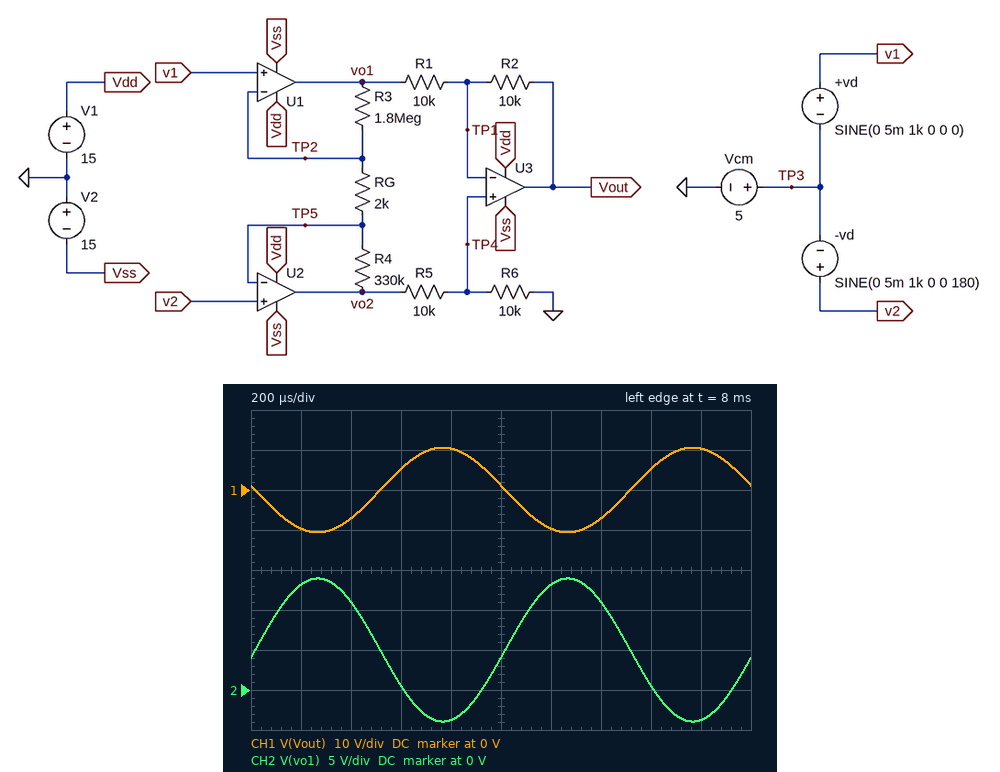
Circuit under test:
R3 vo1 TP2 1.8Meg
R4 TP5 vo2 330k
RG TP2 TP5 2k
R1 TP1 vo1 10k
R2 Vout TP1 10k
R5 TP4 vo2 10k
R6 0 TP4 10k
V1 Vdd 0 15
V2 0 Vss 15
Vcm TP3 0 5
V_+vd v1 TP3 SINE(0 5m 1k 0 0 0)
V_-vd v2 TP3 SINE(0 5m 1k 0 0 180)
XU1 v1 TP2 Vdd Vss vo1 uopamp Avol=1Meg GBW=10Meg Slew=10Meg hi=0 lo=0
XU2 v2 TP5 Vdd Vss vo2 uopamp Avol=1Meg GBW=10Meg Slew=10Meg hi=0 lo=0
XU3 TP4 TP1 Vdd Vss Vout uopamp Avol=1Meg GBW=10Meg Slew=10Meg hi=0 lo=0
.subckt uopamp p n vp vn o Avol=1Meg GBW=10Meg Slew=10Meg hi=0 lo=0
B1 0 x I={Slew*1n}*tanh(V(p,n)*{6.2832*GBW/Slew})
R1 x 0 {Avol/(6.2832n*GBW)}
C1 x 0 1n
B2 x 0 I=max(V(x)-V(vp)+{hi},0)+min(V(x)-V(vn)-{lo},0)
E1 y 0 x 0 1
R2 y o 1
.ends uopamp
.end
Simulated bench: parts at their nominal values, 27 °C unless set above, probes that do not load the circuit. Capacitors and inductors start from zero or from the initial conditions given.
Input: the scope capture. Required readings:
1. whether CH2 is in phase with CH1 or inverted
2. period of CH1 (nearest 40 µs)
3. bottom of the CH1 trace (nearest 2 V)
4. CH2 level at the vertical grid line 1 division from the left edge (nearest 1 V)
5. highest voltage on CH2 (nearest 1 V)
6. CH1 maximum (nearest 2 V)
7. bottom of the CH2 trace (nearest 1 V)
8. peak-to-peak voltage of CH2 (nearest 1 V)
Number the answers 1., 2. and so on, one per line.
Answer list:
1. inverted
2. 1.00 ms
3. -10 V
4. 13 V
5. 14 V
6. 10 V
7. -4 V
8. 18 V
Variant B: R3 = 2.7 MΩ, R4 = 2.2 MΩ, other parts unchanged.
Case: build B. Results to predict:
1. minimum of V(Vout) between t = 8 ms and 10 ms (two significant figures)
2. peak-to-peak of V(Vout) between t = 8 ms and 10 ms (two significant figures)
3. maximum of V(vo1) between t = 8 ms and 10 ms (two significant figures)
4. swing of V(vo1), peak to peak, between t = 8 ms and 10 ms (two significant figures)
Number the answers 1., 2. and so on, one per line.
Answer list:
1. -15 V
2. 30 V
3. 15 V
4. 22 V
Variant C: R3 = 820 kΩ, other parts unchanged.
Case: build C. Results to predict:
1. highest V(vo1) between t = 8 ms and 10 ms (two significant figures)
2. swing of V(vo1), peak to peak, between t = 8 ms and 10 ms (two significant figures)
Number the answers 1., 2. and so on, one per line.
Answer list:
1. 9.1 V
2. 8.2 V
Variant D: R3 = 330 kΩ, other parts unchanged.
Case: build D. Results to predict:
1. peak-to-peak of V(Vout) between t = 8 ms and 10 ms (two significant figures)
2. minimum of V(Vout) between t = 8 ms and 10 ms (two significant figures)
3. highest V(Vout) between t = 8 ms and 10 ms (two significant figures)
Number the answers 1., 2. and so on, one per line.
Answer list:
1. 6.6 V
2. -3.3 V
3. 3.3 V
